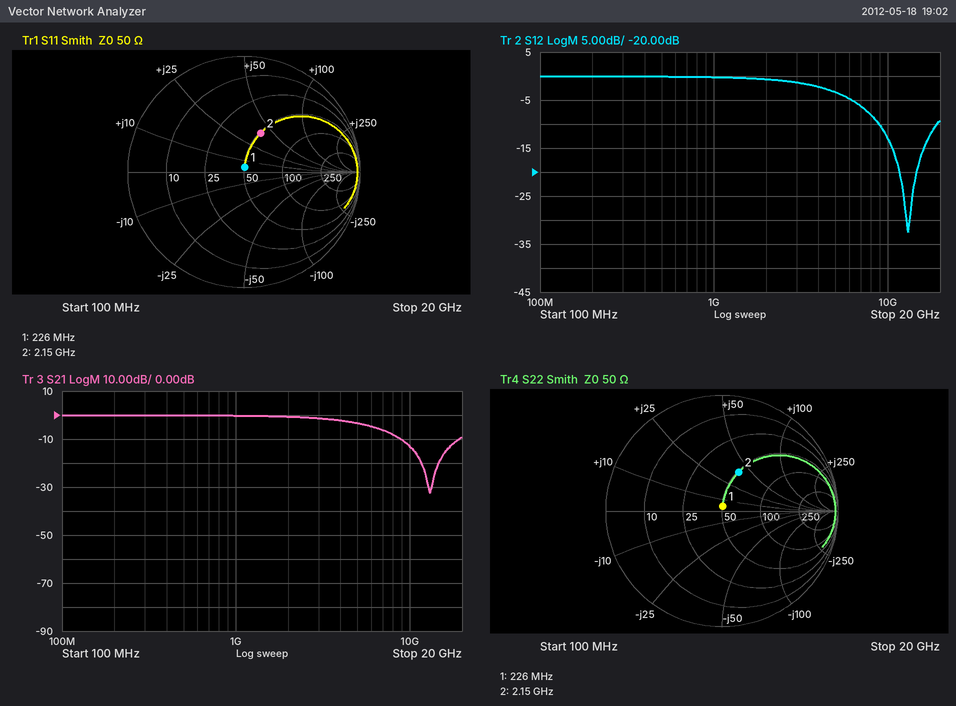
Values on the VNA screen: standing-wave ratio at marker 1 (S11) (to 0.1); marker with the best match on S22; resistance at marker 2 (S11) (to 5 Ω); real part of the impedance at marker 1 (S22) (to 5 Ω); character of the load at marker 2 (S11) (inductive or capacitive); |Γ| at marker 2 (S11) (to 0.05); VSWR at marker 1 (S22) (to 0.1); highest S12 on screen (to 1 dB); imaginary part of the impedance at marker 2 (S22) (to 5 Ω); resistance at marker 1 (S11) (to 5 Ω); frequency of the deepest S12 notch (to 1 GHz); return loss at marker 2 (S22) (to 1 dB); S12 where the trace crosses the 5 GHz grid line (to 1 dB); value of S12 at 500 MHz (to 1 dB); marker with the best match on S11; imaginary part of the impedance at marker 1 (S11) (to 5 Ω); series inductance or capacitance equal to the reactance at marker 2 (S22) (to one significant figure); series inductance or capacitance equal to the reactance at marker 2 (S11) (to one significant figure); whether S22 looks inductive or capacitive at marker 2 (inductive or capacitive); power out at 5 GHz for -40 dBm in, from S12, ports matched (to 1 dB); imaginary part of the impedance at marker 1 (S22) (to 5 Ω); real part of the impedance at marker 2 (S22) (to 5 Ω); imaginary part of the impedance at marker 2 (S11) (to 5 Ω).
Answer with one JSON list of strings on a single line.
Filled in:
["1.1", "marker 1", "50 Ω", "50 Ω", "inductive", "0.35", "1.1", "0 dB", "+40 Ω", "50 Ω", "13 GHz", "9 dB", "-3 dB", "0 dB", "marker 1", "+5 Ω", "3 nH", "3 nH", "inductive", "-43 dBm", "+5 Ω", "50 Ω", "+40 Ω"]
